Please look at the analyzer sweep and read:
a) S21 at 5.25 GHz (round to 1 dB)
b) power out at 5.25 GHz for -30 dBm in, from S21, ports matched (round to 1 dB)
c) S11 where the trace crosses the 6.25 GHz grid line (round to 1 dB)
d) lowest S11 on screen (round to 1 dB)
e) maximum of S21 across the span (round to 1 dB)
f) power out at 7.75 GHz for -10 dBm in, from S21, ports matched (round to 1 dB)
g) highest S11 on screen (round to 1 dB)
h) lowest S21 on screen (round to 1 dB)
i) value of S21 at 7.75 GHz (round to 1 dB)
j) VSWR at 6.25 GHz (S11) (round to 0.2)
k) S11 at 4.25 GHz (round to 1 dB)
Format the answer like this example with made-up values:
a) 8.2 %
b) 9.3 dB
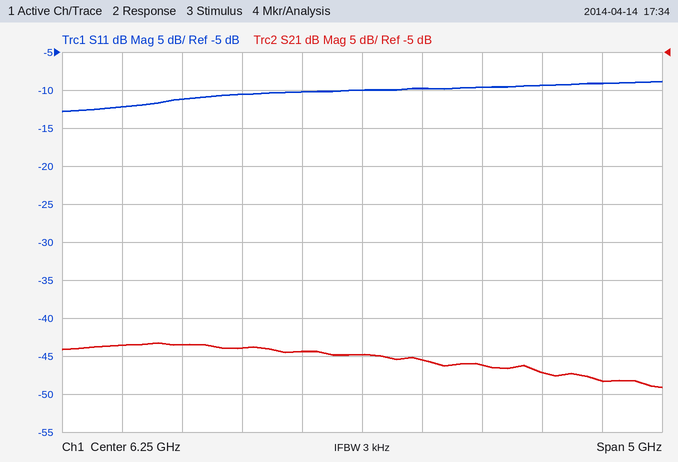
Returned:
a) -44 dB
b) -74 dBm
c) -10 dB
d) -13 dB
e) -43 dB
f) -57 dBm
g) -9 dB
h) -49 dB
i) -47 dB
j) 2.0
k) -12 dB
